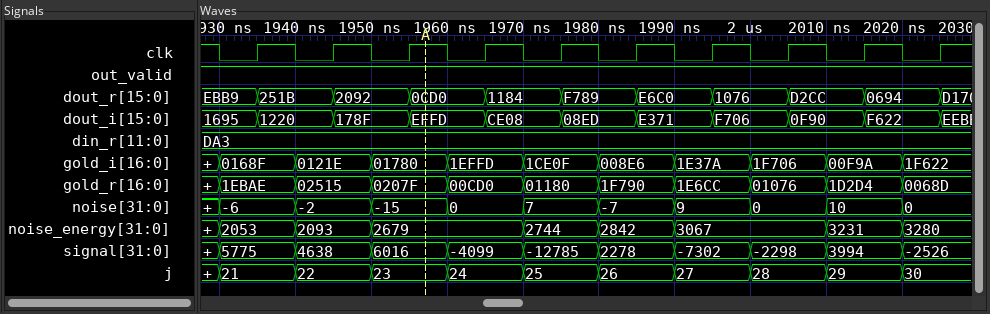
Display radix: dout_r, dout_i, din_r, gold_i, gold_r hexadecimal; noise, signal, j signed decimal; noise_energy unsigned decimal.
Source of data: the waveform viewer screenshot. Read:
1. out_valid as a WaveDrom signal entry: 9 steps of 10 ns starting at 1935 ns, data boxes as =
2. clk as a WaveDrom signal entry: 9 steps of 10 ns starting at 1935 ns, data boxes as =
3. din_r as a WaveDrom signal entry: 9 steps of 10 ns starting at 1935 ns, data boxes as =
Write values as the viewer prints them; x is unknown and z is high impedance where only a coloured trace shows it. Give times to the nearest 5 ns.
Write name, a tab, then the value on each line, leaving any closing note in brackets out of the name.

out_valid as a WaveDrom signal entry: 9 steps of 10 ns starting at 1935 ns, data boxes as =	{name: 'out_valid', wave: '1........'}
clk as a WaveDrom signal entry: 9 steps of 10 ns starting at 1935 ns, data boxes as =	{name: 'clk', wave: 'p........'}
din_r as a WaveDrom signal entry: 9 steps of 10 ns starting at 1935 ns, data boxes as =	{name: 'din_r', wave: '=........', data: 'DA3'}
